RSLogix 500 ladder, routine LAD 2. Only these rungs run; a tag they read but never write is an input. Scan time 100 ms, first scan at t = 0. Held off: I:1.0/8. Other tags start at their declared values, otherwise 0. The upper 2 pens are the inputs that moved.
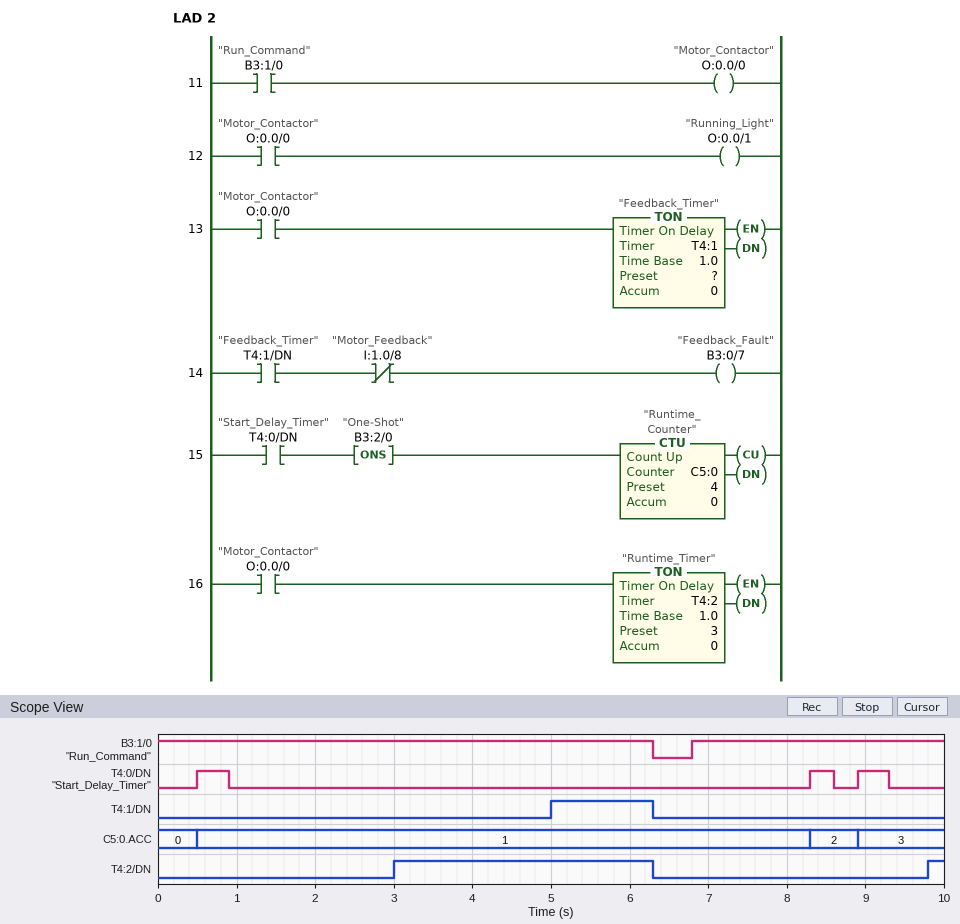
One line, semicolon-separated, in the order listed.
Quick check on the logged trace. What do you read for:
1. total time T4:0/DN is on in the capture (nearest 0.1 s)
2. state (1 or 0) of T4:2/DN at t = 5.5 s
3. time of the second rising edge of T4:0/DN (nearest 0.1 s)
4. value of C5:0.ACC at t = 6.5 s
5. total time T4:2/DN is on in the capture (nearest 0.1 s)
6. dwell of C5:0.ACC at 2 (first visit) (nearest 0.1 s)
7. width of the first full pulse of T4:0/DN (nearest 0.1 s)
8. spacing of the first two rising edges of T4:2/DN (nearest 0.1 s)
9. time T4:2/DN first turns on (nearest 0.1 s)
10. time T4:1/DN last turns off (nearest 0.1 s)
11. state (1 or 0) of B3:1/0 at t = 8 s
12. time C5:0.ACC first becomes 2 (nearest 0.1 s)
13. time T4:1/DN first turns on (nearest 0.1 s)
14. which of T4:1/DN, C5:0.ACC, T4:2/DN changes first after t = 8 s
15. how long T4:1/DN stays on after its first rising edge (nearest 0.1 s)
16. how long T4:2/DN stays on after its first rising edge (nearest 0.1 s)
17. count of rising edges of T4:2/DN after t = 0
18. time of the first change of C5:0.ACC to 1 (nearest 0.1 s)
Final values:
1.1 s; 1; 8.3 s; 1; 3.5 s; 0.6 s; 0.4 s; 6.8 s; 3.0 s; 6.3 s; 1; 8.3 s; 5.0 s; C5:0.ACC; 1.3 s; 3.3 s; 2; 0.5 s
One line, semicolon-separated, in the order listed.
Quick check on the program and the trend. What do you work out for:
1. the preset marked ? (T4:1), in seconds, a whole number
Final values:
5 s
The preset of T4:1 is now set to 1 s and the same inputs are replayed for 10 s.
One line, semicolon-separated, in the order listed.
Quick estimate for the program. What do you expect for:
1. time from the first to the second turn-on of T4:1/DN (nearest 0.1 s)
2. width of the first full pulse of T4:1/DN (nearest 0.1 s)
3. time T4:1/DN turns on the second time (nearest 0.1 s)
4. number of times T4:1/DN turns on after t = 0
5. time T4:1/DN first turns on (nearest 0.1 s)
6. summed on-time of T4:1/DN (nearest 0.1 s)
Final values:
6.8 s; 5.3 s; 7.8 s; 2; 1.0 s; 7.5 s
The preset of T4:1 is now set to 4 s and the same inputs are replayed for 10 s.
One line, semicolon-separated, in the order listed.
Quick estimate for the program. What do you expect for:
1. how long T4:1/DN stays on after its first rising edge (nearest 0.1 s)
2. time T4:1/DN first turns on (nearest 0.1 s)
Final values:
2.3 s; 4.0 s
